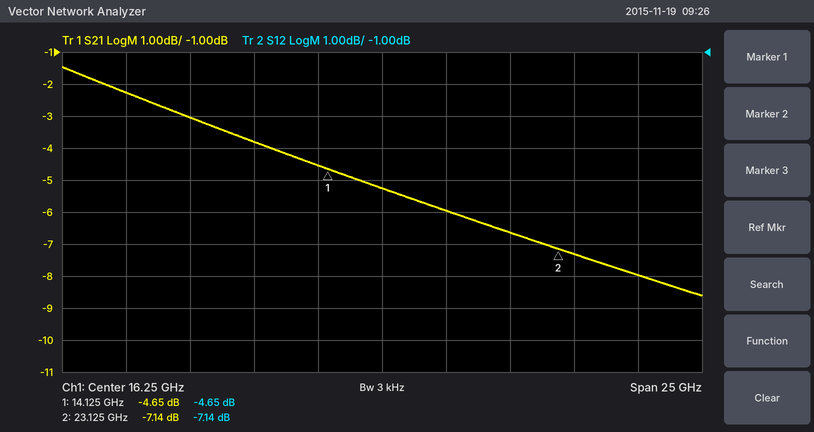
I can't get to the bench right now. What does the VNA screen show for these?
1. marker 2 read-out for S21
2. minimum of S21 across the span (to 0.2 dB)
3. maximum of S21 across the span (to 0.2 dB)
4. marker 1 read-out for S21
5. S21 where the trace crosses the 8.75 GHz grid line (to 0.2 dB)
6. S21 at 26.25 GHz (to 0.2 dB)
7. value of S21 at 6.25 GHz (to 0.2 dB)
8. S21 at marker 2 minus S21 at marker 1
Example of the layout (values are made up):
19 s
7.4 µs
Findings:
-7.14 dB
-8.6 dB
-1.4 dB
-4.65 dB
-3.0 dB
-8.0 dB
-2.2 dB
-2.49 dB
